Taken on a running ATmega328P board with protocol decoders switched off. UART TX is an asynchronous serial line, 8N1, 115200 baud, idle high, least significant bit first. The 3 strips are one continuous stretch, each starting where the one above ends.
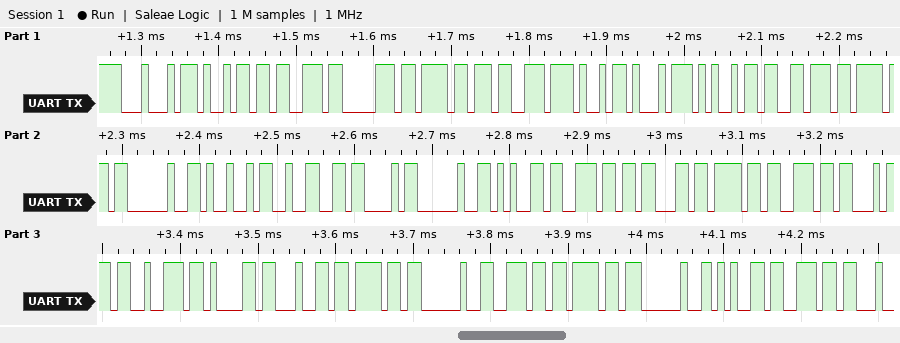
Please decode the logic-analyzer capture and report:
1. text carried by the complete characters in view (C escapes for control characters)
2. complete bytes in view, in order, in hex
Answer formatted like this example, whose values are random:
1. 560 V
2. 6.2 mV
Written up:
1. "Dispositivo I2C encontrado no en"
2. 44 69 73 70 6F 73 69 74 69 76 6F 20 49 32 43 20 65 6E 63 6F 6E 74 72 61 64 6F 20 6E 6F 20 65 6E
